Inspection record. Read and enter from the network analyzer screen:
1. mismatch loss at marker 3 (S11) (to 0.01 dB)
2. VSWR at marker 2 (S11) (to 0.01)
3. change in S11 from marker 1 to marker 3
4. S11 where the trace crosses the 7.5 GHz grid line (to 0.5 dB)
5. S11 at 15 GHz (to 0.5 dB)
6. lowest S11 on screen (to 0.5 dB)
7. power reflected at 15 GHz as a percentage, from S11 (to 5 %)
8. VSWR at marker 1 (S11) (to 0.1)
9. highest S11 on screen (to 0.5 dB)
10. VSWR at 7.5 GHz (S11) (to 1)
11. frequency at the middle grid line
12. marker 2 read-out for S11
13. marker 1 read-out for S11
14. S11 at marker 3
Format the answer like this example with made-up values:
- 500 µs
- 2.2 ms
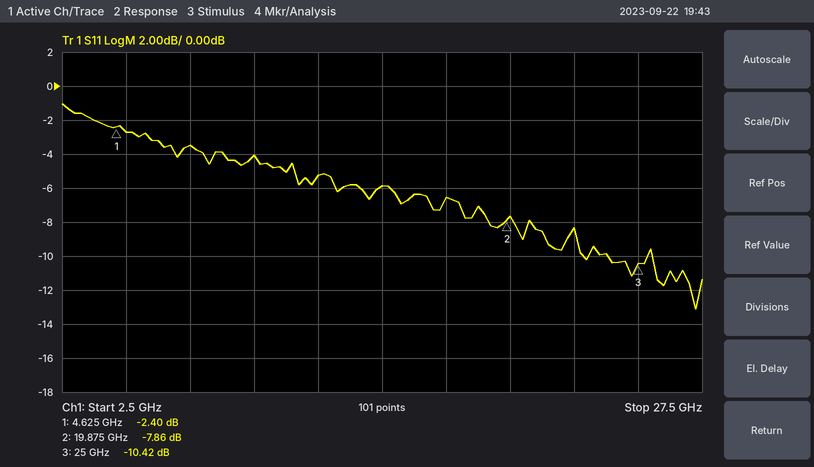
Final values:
- 0.41 dB
- 2.36
- -8.02 dB
- -3.5 dB
- -6.0 dB
- -13.0 dB
- 25 %
- 7.3
- -1.0 dB
- 5
- 15 GHz
- -7.86 dB
- -2.40 dB
- -10.42 dB
